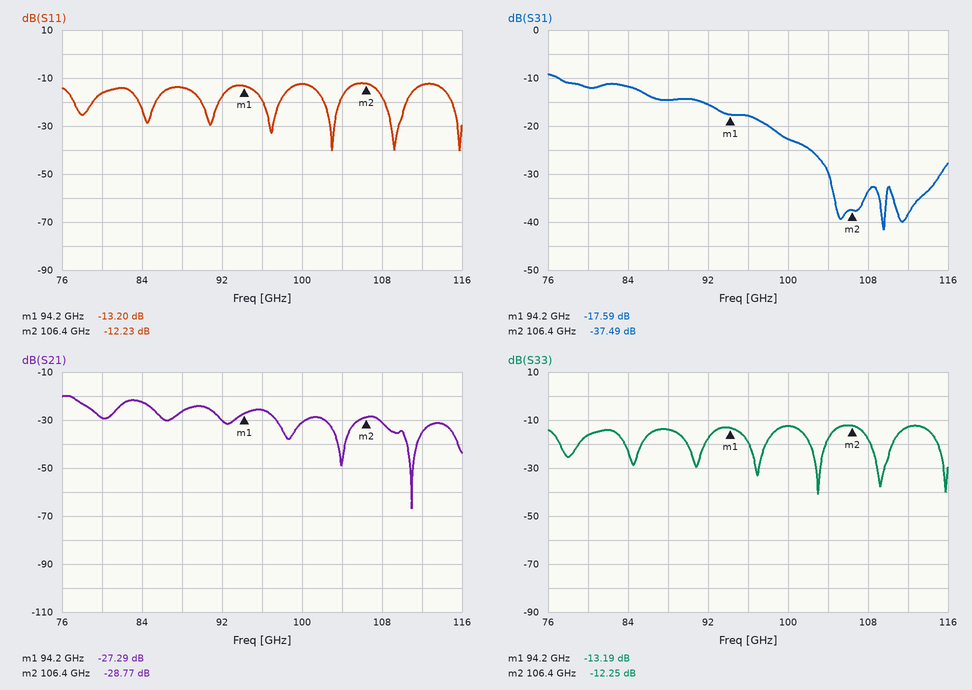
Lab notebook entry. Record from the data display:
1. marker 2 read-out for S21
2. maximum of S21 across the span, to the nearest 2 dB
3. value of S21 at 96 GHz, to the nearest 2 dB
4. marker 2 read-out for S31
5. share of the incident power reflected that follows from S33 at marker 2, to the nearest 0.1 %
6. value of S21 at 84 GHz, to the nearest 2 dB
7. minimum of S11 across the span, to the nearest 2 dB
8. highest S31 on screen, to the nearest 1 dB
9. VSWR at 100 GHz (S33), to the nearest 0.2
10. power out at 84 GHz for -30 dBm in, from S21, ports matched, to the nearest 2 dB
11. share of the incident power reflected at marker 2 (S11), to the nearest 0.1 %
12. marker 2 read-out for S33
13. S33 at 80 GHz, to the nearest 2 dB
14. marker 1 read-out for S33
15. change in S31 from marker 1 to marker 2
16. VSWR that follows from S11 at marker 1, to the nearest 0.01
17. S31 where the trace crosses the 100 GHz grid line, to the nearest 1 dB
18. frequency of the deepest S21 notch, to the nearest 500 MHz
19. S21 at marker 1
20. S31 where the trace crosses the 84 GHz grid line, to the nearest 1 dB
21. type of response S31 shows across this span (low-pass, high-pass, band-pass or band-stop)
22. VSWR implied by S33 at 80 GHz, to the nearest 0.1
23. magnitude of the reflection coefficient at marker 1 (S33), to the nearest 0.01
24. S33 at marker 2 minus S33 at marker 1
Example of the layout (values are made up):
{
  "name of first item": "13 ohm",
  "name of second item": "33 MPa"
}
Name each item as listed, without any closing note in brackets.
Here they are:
{
  "marker 2 read-out for S21": "-28.77 dB",
  "maximum of S21 across the span, to the nearest 2 dB": "-20 dB",
  "value of S21 at 96 GHz, to the nearest 2 dB": "-26 dB",
  "marker 2 read-out for S31": "-37.49 dB",
  "share of the incident power reflected that follows from S33 at marker 2, to the nearest 0.1 %": "6.0 %",
  "value of S21 at 84 GHz, to the nearest 2 dB": "-22 dB",
  "minimum of S11 across the span, to the nearest 2 dB": "-40 dB",
  "highest S31 on screen, to the nearest 1 dB": "-9 dB",
  "VSWR at 100 GHz (S33), to the nearest 0.2": "1.6",
  "power out at 84 GHz for -30 dBm in, from S21, ports matched, to the nearest 2 dB": "-52 dBm",
  "share of the incident power reflected at marker 2 (S11), to the nearest 0.1 %": "6.0 %",
  "marker 2 read-out for S33": "-12.25 dB",
  "S33 at 80 GHz, to the nearest 2 dB": "-16 dB",
  "marker 1 read-out for S33": "-13.19 dB",
  "change in S31 from marker 1 to marker 2": "-19.90 dB",
  "VSWR that follows from S11 at marker 1, to the nearest 0.01": "1.56",
  "S31 where the trace crosses the 100 GHz grid line, to the nearest 1 dB": "-23 dB",
  "frequency of the deepest S21 notch, to the nearest 500 MHz": "111.0 GHz",
  "S21 at marker 1": "-27.29 dB",
  "S31 where the trace crosses the 84 GHz grid line, to the nearest 1 dB": "-12 dB",
  "type of response S31 shows across this span": "low-pass",
  "VSWR implied by S33 at 80 GHz, to the nearest 0.1": "1.4",
  "magnitude of the reflection coefficient at marker 1 (S33), to the nearest 0.01": "0.22",
  "S33 at marker 2 minus S33 at marker 1": "0.94 dB"
}
